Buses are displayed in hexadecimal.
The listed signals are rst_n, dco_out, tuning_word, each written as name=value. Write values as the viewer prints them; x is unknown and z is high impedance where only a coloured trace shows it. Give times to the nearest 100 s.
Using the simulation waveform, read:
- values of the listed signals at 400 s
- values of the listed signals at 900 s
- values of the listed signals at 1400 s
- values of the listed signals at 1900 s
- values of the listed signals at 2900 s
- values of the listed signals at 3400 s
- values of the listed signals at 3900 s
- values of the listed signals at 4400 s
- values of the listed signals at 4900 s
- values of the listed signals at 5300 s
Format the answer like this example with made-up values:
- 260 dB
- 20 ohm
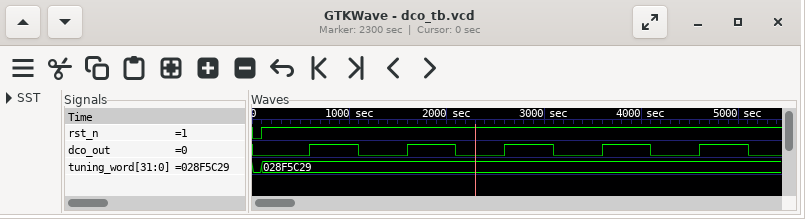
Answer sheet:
- rst_n=1, dco_out=0, tuning_word=028F5C29
- rst_n=1, dco_out=1, tuning_word=028F5C29
- rst_n=1, dco_out=0, tuning_word=028F5C29
- rst_n=1, dco_out=1, tuning_word=028F5C29
- rst_n=1, dco_out=1, tuning_word=028F5C29
- rst_n=1, dco_out=0, tuning_word=028F5C29
- rst_n=1, dco_out=1, tuning_word=028F5C29
- rst_n=1, dco_out=0, tuning_word=028F5C29
- rst_n=1, dco_out=1, tuning_word=028F5C29
- rst_n=1, dco_out=0, tuning_word=028F5C29
